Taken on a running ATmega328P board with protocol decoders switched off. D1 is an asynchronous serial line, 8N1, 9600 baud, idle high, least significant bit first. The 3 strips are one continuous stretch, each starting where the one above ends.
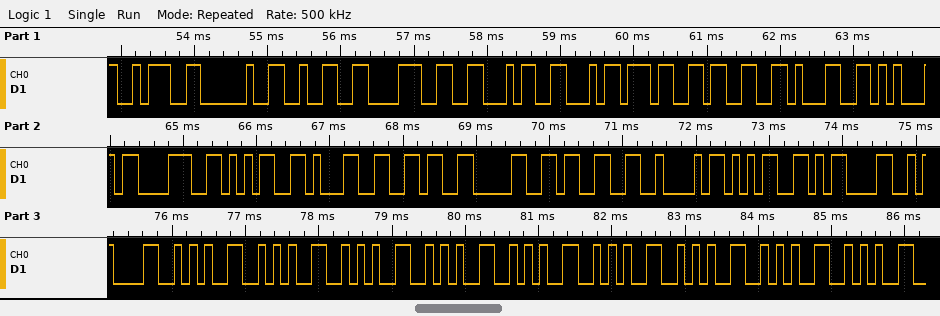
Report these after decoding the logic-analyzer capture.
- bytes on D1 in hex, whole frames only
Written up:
3A 20 32 38 46 46 37 33 31 45 38 35 31 36 30 33 42 35 0D 0A 2A 2A 2A 2A 2A 2A 2A 2A 2A
